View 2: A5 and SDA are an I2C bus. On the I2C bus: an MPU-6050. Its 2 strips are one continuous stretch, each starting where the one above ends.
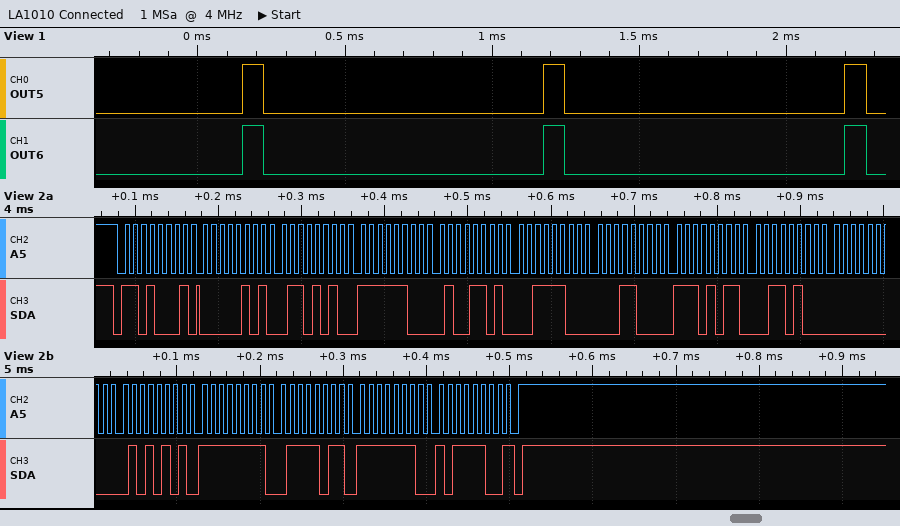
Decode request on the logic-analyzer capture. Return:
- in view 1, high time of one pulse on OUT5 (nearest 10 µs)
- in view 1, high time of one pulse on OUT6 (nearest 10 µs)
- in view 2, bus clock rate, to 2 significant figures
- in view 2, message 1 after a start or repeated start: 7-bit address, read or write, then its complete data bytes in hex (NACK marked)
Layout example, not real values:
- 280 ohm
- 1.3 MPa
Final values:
- 70 µs
- 70 µs
- 100 kHz
- 0x68 read: 05 6A FC 4D 3C 18 EB 34 00 55 FF 7B FE BC NACK
